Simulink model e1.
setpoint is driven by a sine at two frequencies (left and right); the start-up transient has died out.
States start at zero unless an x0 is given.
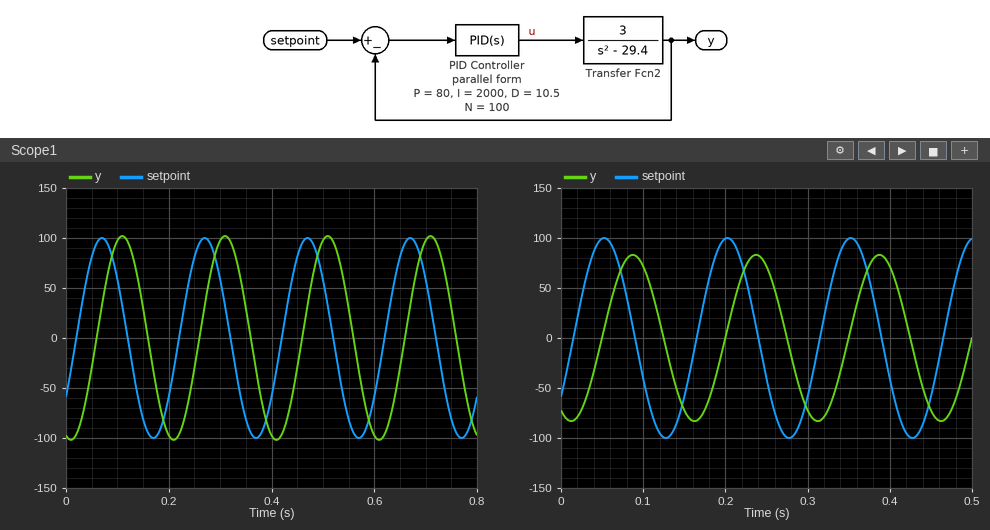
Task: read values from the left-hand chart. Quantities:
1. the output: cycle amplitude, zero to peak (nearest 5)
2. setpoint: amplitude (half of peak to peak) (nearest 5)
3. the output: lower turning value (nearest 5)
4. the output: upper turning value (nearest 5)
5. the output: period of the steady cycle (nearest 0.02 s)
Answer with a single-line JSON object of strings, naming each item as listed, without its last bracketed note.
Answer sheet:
{"the output: cycle amplitude, zero to peak": "100", "setpoint: amplitude (half of peak to peak)": "100", "the output: lower turning value": "-100", "the output: upper turning value": "100", "the output: period of the steady cycle": "0.20 s"}
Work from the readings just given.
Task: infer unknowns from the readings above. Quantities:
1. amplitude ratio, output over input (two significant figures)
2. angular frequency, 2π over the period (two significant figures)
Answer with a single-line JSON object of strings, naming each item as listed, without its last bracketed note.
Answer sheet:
{"amplitude ratio, output over input": "1.0", "angular frequency, 2π over the period": "31 rad/s"}
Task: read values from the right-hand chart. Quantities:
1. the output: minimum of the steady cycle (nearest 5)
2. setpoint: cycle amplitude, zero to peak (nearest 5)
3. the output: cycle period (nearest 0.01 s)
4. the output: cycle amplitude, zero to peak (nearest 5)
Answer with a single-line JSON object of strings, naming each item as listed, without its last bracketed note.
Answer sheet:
{"the output: minimum of the steady cycle": "-85", "setpoint: cycle amplitude, zero to peak": "100", "the output: cycle period": "0.15 s", "the output: cycle amplitude, zero to peak": "85"}
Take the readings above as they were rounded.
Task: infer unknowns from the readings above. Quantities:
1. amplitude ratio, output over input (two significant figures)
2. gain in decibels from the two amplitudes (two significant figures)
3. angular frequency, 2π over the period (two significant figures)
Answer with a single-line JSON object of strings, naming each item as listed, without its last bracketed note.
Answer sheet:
{"amplitude ratio, output over input": "0.85", "gain in decibels from the two amplitudes": "-1.4 dB", "angular frequency, 2π over the period": "42 rad/s"}
